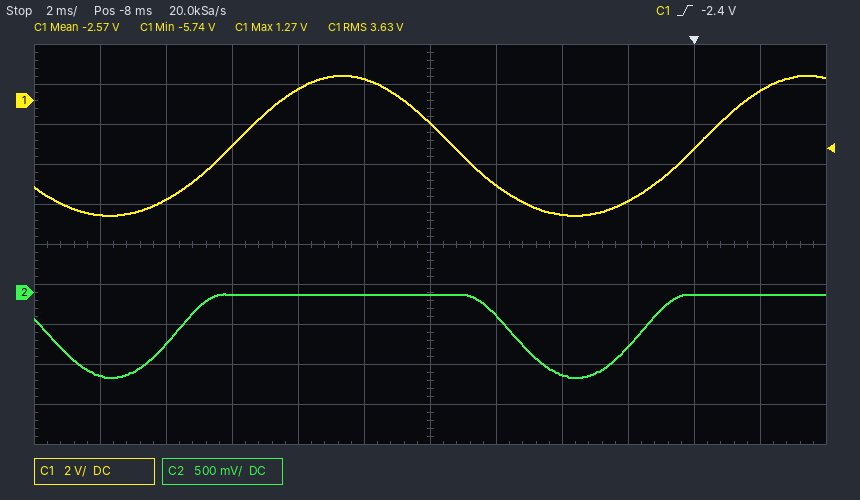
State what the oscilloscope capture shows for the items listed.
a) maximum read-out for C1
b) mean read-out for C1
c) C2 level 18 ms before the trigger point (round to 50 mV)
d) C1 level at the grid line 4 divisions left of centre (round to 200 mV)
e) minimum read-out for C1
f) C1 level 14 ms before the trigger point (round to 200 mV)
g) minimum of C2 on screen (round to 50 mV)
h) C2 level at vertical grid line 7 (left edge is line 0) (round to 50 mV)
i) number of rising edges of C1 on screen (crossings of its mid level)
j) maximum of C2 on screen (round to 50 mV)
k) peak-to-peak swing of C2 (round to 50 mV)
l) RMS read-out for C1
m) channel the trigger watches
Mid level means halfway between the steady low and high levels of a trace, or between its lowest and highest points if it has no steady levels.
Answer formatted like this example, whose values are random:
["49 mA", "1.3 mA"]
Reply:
["1.27 V", "-2.57 V", "-1.05 V", "-5.0 V", "-5.74 V", "-2.2 V", "-1.05 V", "-300 mV", "2", "0 mV", "1.05 V", "3.63 V", "C1"]
